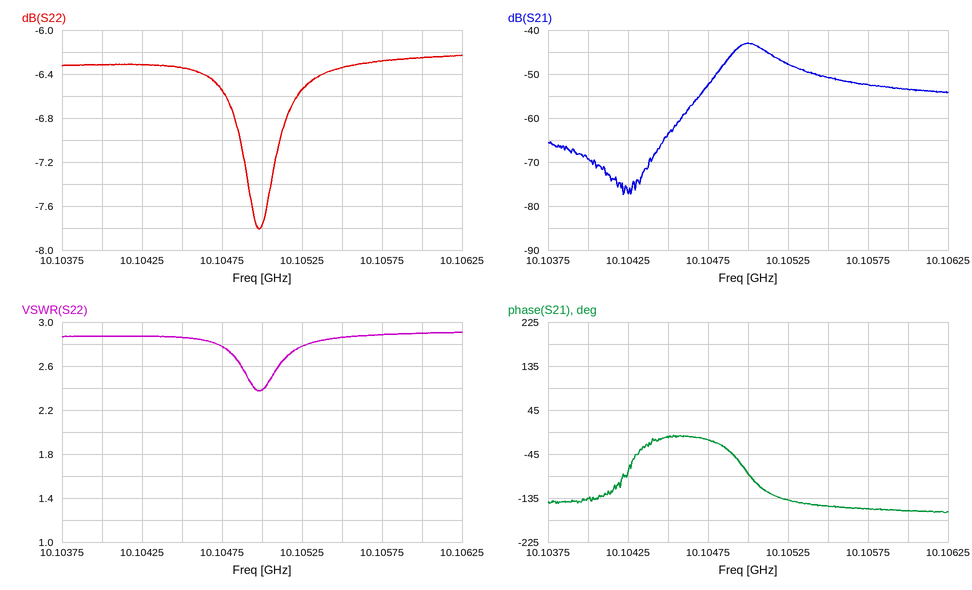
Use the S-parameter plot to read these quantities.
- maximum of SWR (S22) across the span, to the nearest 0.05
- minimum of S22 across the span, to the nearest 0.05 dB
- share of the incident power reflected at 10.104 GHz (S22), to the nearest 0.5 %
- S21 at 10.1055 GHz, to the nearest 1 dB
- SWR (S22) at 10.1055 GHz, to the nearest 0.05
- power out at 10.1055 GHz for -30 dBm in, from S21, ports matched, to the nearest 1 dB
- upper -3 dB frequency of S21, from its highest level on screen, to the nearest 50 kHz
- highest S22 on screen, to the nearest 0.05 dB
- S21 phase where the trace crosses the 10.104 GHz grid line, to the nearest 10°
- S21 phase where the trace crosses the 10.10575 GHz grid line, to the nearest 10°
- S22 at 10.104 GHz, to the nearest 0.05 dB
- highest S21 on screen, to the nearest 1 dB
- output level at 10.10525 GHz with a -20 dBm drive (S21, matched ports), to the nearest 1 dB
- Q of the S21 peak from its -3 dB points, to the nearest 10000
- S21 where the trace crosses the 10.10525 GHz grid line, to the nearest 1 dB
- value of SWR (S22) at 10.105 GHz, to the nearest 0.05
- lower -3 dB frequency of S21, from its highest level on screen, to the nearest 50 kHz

2.90
-7.80 dB
23.5 %
-51 dB
2.85
-81 dBm
10.10515 GHz
-6.25 dB
-140°
-160°
-6.30 dB
-43 dB
-68 dBm
40000
-48 dB
2.40
10.10490 GHz
